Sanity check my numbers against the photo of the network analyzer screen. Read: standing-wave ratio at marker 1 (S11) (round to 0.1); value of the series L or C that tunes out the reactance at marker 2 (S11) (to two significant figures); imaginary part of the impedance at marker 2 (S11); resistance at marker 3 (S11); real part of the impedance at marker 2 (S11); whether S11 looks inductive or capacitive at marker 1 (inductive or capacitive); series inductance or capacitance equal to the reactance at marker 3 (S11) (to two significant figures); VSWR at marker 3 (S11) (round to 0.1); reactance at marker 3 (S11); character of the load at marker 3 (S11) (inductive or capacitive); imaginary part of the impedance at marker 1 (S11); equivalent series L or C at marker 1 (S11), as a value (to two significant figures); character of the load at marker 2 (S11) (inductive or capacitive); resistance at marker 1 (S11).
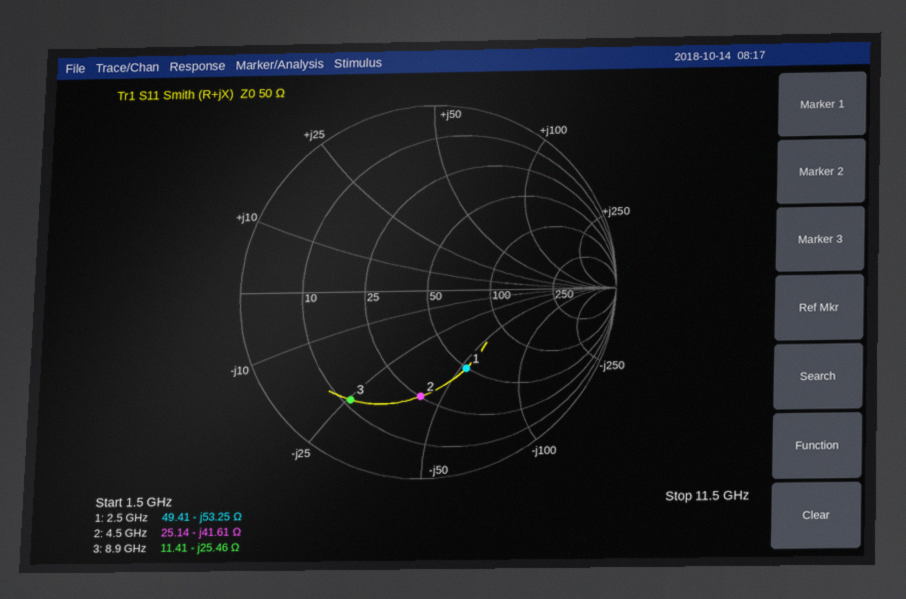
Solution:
2.8
1.5 nH
-41.61 Ω
11.41 Ω
25.14 Ω
capacitive
700 fF
5.6
-25.46 Ω
capacitive
-53.25 Ω
1.2 pF
capacitive
49.41 Ω
